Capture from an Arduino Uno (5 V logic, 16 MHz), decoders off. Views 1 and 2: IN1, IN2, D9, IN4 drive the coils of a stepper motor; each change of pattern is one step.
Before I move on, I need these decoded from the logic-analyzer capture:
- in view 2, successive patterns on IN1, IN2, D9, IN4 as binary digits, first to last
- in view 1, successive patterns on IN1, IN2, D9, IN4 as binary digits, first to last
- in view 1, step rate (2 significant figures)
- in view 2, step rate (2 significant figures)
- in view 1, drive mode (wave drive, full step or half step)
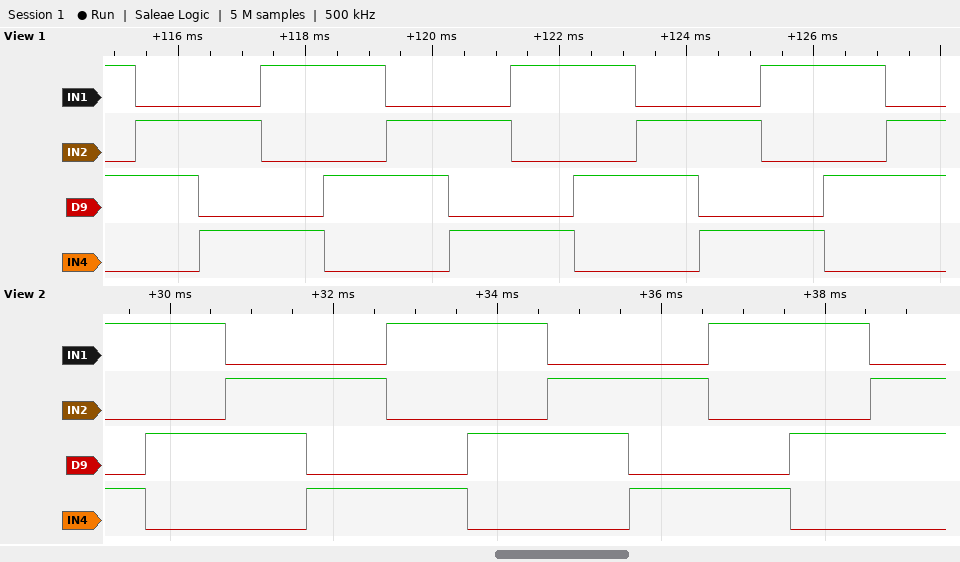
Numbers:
1001 1010 0110 0101 1001 1010 0110 0101 1001 1010 0110
1010 0110 0101 1001 1010 0110 0101 1001 1010 0110 0101 1001 1010 0110
1000 steps/s
1000 steps/s
full step
